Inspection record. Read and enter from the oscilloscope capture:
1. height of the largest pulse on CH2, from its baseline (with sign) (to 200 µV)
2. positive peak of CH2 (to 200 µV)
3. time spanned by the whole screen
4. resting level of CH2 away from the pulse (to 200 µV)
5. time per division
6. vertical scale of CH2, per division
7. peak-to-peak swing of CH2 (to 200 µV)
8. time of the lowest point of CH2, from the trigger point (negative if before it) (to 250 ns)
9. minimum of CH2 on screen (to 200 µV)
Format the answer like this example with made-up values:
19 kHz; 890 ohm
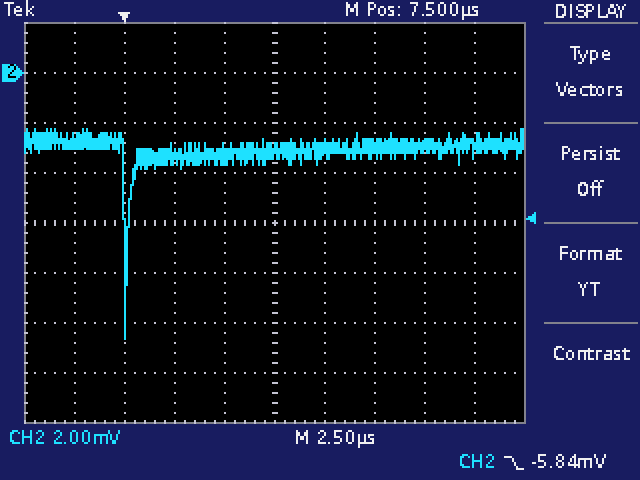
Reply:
-7.6 mV; -2.2 mV; 25 µs; -3.0 mV; 2.5 µs; 2 mV; 8.4 mV; 0.00 µs; -10.6 mV
